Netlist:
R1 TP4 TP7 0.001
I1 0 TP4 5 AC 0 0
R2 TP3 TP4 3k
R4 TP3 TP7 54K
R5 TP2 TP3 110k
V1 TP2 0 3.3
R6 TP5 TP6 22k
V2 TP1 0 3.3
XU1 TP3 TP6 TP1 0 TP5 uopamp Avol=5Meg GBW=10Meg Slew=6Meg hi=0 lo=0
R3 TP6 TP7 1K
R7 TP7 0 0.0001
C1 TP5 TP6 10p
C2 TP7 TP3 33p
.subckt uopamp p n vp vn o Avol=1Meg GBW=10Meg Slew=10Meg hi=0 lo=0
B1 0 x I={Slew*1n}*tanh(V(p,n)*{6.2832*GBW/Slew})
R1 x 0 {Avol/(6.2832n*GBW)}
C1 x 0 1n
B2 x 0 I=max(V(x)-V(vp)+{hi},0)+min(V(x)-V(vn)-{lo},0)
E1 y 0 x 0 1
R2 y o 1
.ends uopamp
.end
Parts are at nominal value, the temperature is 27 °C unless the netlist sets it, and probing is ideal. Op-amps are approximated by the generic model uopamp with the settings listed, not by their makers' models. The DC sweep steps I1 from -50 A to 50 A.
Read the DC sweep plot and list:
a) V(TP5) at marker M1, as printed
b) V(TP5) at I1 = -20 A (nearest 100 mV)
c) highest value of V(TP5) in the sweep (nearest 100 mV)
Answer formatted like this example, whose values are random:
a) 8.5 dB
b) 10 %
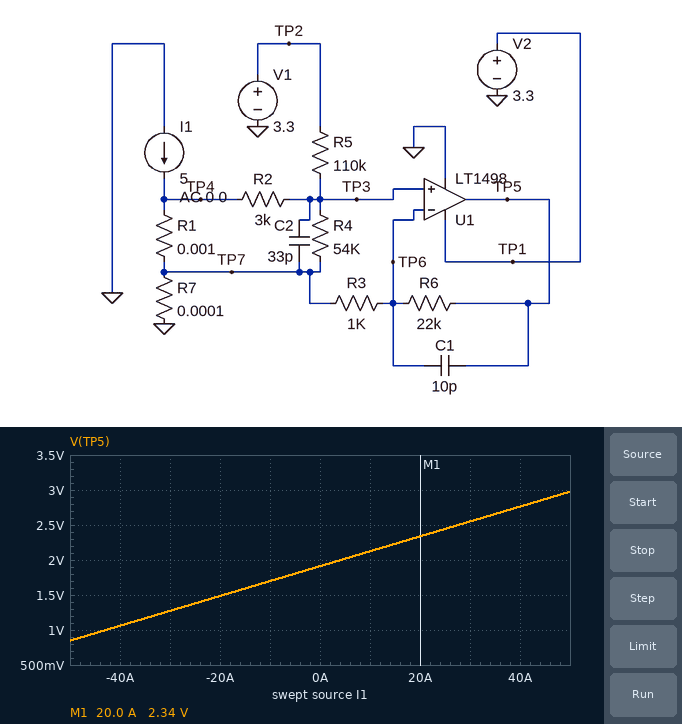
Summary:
a) 2.34 V
b) 1.5 V
c) 3.0 V
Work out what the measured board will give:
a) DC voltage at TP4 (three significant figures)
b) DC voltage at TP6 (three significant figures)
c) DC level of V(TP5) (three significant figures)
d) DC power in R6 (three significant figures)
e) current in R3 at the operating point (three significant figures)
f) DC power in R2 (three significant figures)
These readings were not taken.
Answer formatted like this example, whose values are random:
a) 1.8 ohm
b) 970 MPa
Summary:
a) 5.50 mV
b) 88.2 mV
c) 2.02 V
d) 169 µW
e) 87.7 µA
f) 2.28 µW
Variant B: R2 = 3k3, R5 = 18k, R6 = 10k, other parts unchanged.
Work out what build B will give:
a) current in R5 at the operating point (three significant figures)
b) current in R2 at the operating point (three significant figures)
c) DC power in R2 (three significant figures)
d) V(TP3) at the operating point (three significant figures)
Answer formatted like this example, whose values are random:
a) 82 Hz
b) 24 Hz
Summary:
a) 156 µA
b) 147 µA
c) 71.3 µW
d) 491 mV
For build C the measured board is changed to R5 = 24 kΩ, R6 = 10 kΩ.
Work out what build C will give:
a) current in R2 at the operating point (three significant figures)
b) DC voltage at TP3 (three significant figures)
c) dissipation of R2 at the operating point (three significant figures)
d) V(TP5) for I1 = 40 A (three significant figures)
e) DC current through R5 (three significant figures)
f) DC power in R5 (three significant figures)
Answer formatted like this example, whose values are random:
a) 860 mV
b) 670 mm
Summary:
a) 116 µA
b) 354 mV
c) 40.5 µW
d) 3.30 V
e) 123 µA
f) 362 µW
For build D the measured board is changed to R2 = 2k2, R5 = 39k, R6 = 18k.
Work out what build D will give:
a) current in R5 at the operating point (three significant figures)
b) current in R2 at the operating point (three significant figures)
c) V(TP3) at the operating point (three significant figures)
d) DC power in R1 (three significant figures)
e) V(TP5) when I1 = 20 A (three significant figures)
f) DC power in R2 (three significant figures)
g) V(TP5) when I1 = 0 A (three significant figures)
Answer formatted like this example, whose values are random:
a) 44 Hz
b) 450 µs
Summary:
a) 80.1 µA
b) 76.9 µA
c) 175 mV
d) 25.0 mW
e) 3.30 V
f) 13.0 µW
g) 3.22 V
